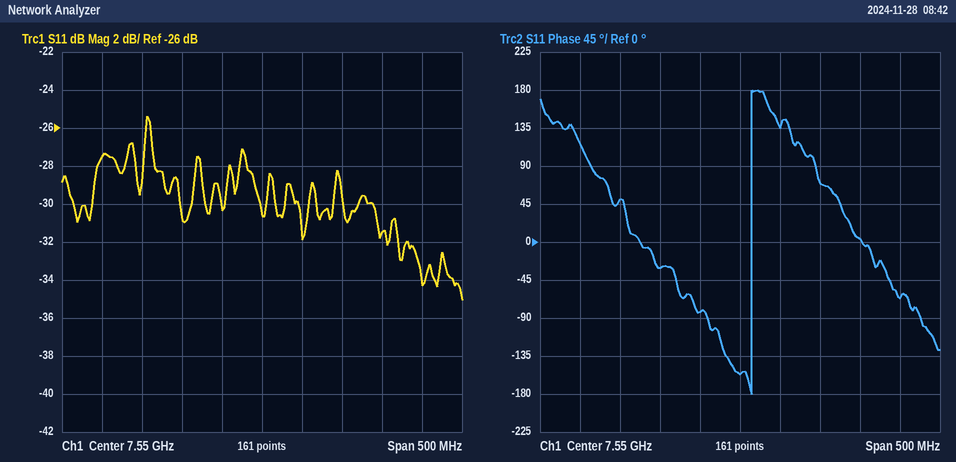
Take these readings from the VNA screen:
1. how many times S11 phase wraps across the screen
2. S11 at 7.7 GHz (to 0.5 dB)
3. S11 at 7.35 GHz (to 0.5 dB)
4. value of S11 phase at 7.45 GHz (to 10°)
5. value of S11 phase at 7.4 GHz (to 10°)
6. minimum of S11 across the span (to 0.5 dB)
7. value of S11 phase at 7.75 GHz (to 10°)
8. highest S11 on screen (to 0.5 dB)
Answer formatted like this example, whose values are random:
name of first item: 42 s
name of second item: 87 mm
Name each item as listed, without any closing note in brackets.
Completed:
how many times S11 phase wraps across the screen: 1
S11 at 7.7 GHz: -31.5 dB
S11 at 7.35 GHz: -27.5 dB
value of S11 phase at 7.45 GHz: -30°
value of S11 phase at 7.4 GHz: 50°
minimum of S11 across the span: -35.0 dB
value of S11 phase at 7.75 GHz: -70°
highest S11 on screen: -25.5 dB
